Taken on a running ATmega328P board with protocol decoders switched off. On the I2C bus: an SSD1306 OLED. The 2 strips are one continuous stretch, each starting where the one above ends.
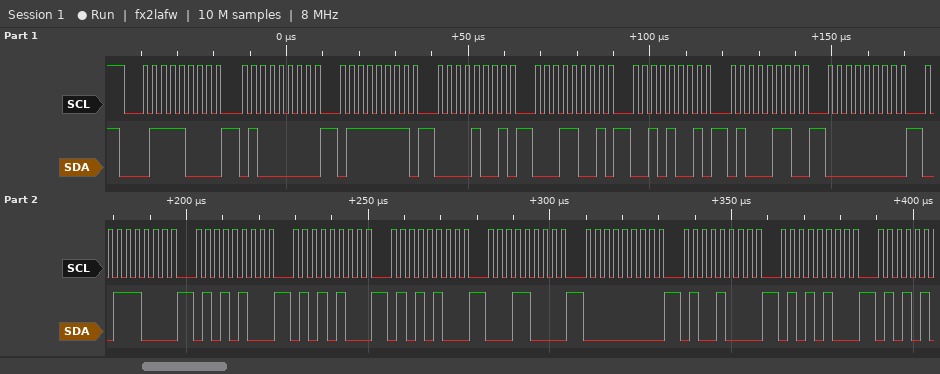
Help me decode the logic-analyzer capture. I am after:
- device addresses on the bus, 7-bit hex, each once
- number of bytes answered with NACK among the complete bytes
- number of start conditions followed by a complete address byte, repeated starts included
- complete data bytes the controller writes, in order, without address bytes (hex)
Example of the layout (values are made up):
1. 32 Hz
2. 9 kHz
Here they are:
1. 0x3C
2. 0
3. 1
4. 40 7F 09 19 29 46 00 38 54 54 54 18 00 48 54
